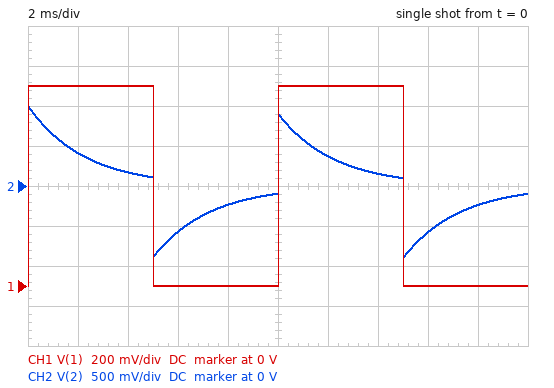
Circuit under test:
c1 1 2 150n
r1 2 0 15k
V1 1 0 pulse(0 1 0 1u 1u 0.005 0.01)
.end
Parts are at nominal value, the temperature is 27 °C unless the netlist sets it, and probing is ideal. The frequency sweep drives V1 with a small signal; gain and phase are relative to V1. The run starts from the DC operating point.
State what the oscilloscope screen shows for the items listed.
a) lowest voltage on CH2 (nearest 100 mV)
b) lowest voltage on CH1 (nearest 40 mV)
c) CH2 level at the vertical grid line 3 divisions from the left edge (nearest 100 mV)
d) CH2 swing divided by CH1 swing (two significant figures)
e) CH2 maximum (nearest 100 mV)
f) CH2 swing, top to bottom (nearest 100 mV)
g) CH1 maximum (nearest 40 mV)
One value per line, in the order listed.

-900 mV
0 V
-600 mV
1.9
1.0 V
1.9 V
1.00 V
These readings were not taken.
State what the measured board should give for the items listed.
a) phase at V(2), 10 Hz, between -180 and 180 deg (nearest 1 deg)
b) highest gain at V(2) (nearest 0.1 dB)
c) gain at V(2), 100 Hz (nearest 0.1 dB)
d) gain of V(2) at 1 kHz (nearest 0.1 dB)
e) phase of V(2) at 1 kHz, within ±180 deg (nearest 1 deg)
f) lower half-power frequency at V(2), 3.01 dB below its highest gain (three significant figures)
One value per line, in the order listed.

82 deg
0 dB
-1.8 dB
0 dB
4 deg
70.7 Hz
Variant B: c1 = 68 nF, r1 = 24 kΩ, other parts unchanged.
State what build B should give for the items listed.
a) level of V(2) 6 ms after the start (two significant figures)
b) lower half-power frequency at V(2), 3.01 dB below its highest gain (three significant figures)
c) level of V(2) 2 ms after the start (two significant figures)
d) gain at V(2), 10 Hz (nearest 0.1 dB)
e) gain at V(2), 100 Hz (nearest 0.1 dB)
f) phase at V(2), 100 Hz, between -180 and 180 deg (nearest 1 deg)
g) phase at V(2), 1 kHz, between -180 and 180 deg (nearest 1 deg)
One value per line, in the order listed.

-520 mV
97.5 Hz
290 mV
-19.8 dB
-2.9 dB
44 deg
6 deg
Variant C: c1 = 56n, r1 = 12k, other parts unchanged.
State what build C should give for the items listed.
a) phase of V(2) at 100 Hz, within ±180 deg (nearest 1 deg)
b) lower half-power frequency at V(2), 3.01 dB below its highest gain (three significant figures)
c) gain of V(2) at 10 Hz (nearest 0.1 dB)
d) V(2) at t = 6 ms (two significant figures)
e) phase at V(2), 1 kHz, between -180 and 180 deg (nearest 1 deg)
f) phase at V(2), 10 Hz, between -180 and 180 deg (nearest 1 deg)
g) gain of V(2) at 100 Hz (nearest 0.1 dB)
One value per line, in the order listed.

67 deg
237 Hz
-27.5 dB
-230 mV
13 deg
88 deg
-8.2 dB
